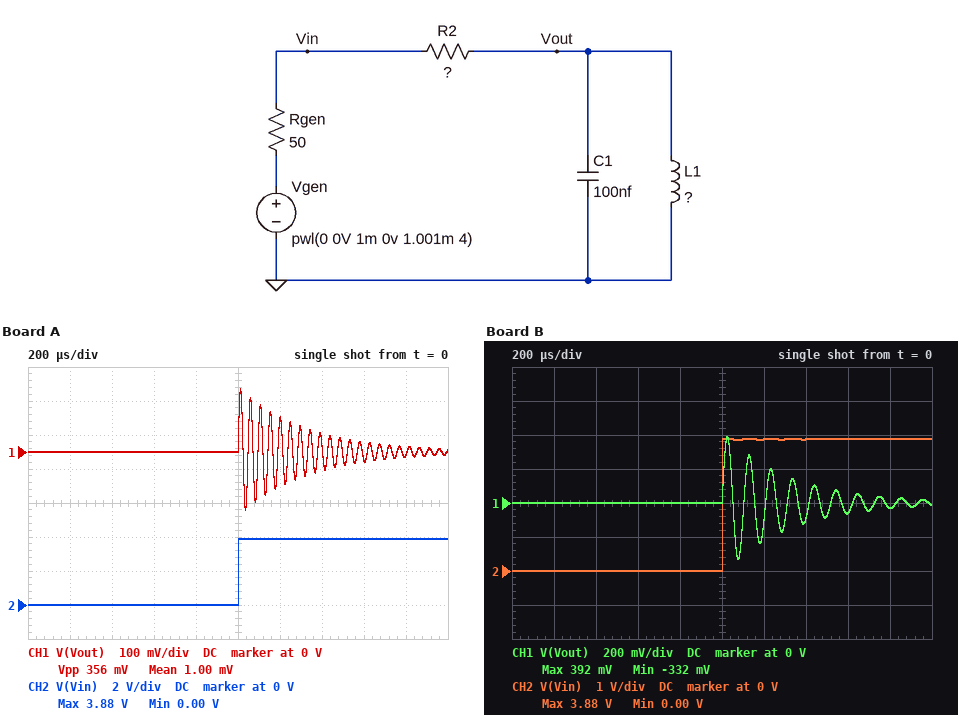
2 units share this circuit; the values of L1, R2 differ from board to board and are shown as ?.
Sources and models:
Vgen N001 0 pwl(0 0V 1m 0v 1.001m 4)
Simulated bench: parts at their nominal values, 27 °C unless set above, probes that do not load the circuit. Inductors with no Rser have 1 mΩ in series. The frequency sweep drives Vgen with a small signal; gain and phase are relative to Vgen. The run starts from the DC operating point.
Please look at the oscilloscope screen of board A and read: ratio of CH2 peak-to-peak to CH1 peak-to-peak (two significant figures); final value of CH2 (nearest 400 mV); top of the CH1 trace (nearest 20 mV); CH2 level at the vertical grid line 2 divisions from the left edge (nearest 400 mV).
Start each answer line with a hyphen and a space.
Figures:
- 11
- 4.0 V
- 180 mV
- 0 V
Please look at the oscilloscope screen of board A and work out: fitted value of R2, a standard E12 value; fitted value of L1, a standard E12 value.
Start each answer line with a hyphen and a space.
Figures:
- 1.5 kΩ
- 560 µH
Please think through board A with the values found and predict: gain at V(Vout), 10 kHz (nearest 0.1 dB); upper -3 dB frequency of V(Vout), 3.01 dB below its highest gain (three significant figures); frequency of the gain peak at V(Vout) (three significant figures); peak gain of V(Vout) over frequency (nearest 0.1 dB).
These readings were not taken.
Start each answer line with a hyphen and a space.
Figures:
- -30.7 dB
- 21.8 kHz
- 21.3 kHz
- 0 dB
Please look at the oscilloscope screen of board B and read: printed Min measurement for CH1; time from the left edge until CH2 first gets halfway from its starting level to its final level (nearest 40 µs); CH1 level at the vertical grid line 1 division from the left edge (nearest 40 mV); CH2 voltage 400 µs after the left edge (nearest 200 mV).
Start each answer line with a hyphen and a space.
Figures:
- -332 mV
- 1.00 ms
- 0 V
- 0 V
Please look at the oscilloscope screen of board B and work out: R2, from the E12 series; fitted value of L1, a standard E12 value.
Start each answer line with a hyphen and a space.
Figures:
- 1.5 kΩ
- 2.7 mH
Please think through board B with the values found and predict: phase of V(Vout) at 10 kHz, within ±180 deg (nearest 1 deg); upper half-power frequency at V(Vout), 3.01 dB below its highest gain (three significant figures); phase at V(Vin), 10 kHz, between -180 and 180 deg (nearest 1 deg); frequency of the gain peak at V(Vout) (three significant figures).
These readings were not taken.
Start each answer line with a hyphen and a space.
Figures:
- -31 deg
- 10.2 kHz
- -1 deg
- 9.69 kHz
